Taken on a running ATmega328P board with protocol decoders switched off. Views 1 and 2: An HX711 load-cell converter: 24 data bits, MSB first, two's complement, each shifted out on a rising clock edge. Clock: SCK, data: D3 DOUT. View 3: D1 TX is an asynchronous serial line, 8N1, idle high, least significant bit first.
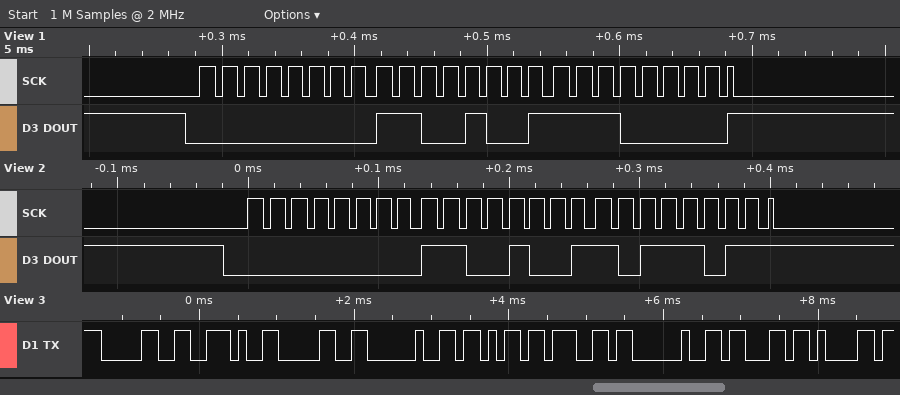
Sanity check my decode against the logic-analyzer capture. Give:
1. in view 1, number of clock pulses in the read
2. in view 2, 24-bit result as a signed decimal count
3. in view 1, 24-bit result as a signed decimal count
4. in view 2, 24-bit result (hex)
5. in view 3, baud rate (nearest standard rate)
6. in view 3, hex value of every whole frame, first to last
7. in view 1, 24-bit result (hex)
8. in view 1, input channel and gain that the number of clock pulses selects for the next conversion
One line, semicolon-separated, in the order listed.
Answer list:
25; 51643; 51680; 0x00C9BB; 9600 baud; 30 2E 30 20 6B 67 20 63 61; 0x00C9E0; channel A, gain 128
